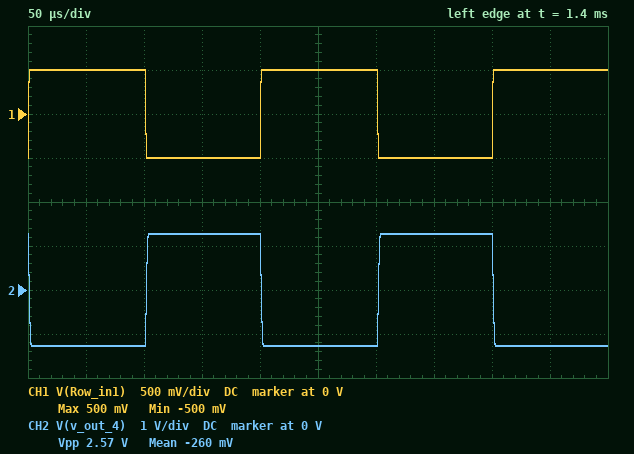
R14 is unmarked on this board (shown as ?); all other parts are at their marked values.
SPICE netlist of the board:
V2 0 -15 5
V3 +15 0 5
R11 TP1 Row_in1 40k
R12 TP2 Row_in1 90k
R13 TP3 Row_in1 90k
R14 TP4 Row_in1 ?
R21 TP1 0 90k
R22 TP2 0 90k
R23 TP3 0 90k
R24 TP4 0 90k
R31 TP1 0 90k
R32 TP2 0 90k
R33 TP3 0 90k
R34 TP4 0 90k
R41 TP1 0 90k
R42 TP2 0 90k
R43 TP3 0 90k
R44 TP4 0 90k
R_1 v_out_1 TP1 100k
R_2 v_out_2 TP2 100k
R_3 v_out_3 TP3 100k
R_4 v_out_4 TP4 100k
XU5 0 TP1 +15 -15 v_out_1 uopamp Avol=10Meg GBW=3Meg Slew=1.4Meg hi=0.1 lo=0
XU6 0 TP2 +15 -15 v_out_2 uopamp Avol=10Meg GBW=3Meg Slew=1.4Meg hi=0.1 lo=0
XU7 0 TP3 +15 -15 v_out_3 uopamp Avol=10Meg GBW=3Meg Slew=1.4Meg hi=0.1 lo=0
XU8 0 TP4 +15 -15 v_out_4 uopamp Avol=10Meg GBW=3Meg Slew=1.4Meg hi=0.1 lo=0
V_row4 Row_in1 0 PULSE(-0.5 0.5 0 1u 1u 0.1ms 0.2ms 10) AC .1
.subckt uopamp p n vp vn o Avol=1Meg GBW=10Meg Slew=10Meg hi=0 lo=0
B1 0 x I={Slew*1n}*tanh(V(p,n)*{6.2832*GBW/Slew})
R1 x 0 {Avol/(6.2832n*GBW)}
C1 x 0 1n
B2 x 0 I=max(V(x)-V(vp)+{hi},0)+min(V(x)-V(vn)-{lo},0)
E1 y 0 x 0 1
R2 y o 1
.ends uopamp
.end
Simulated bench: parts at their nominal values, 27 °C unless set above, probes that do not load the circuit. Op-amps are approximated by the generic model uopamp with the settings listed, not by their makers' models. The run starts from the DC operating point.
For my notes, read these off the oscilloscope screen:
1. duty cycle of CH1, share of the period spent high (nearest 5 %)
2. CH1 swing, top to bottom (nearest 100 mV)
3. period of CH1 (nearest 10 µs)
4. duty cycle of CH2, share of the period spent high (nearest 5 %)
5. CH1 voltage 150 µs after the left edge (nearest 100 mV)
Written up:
50 %
1.0 V
200 µs
50 %
-500 mV
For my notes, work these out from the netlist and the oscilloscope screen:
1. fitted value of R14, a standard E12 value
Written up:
39 kΩ
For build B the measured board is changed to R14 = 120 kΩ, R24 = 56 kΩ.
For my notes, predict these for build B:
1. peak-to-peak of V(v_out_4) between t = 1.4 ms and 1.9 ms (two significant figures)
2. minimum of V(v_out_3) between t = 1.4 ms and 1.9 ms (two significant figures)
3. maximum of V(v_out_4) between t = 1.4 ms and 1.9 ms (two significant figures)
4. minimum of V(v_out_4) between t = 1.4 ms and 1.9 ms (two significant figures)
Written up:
830 mV
-560 mV
420 mV
-420 mV
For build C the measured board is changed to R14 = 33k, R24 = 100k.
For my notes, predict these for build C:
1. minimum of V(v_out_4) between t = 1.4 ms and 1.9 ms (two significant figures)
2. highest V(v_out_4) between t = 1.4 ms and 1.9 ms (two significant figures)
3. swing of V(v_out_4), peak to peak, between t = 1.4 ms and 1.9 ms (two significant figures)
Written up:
-1.5 V
1.5 V
3.0 V
